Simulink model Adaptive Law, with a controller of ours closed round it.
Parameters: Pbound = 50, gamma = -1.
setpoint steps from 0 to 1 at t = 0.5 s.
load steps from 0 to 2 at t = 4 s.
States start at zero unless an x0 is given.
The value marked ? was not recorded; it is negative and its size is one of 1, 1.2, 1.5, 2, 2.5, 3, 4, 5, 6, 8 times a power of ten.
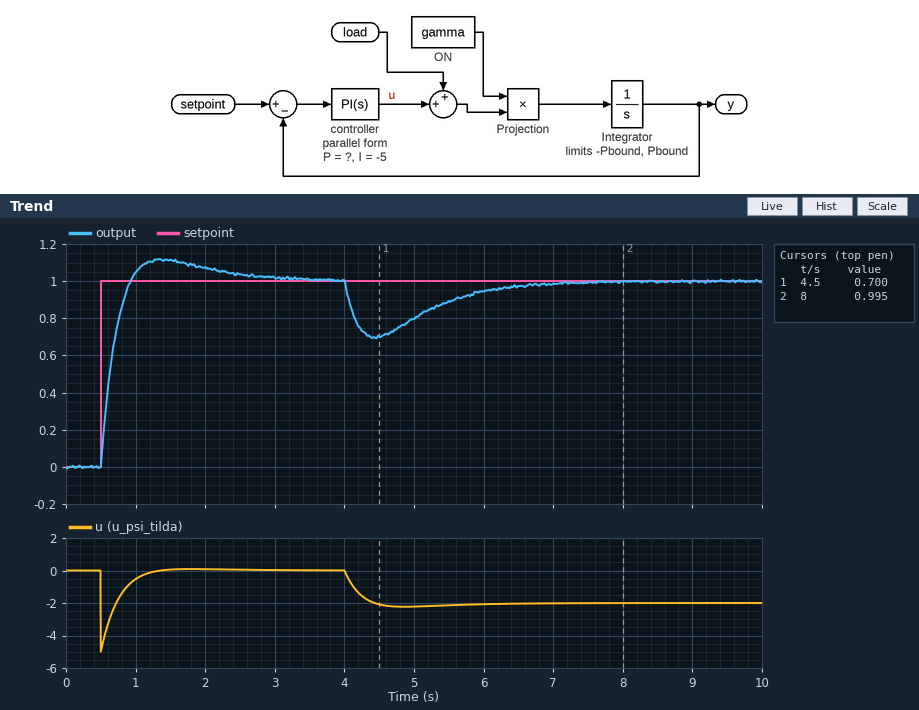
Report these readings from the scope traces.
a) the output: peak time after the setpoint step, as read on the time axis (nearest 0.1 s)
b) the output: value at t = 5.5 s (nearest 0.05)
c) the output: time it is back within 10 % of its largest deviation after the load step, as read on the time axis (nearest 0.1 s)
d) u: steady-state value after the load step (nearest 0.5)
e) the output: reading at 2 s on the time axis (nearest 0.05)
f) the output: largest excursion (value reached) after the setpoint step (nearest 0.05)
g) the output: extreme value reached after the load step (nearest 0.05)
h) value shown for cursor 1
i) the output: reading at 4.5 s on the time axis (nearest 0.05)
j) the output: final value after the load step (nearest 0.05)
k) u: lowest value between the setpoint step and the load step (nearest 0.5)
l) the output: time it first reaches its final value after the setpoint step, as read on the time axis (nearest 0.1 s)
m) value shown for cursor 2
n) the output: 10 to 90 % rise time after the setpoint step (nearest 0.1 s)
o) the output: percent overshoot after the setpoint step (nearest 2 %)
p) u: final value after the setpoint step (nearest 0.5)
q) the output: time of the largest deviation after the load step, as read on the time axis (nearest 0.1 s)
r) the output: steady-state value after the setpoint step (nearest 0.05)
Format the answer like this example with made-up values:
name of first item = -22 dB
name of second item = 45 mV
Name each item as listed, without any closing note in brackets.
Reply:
the output: peak time after the setpoint step, as read on the time axis = 1.4 s
the output: value at t = 5.5 s = 0.90
the output: time it is back within 10 % of its largest deviation after the load step, as read on the time axis = 6.4 s
u: steady-state value after the load step = -2.0
the output: reading at 2 s on the time axis = 1.05
the output: largest excursion (value reached) after the setpoint step = 1.10
the output: extreme value reached after the load step = 0.70
value shown for cursor 1 = 0.700
the output: reading at 4.5 s on the time axis = 0.70
the output: final value after the load step = 1.00
u: lowest value between the setpoint step and the load step = -5.0
the output: time it first reaches its final value after the setpoint step, as read on the time axis = 0.9 s
value shown for cursor 2 = 0.995
the output: 10 to 90 % rise time after the setpoint step = 0.3 s
the output: percent overshoot after the setpoint step = 12 %
u: final value after the setpoint step = 0.0
the output: time of the largest deviation after the load step, as read on the time axis = 4.4 s
the output: steady-state value after the setpoint step = 1.00
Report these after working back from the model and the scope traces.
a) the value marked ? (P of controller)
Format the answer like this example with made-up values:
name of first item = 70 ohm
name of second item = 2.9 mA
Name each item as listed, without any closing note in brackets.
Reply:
the value marked ? = -5
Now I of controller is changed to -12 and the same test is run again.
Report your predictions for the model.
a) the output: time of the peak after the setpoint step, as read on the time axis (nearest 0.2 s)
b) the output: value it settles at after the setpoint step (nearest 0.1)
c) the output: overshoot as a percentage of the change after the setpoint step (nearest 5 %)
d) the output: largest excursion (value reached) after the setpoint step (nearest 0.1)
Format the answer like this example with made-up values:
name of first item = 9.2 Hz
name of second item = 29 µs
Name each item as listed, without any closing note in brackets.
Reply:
the output: time of the peak after the setpoint step, as read on the time axis = 1.2 s
the output: value it settles at after the setpoint step = 1.0
the output: overshoot as a percentage of the change after the setpoint step = 20 %
the output: largest excursion (value reached) after the setpoint step = 1.2
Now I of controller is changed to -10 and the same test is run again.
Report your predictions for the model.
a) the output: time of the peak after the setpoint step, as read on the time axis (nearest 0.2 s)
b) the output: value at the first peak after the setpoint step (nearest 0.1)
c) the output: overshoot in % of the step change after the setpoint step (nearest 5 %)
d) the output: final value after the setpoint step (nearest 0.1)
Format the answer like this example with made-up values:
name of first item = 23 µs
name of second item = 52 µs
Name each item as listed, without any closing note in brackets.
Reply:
the output: time of the peak after the setpoint step, as read on the time axis = 1.2 s
the output: value at the first peak after the setpoint step = 1.2
the output: overshoot in % of the step change after the setpoint step = 20 %
the output: final value after the setpoint step = 1.0
